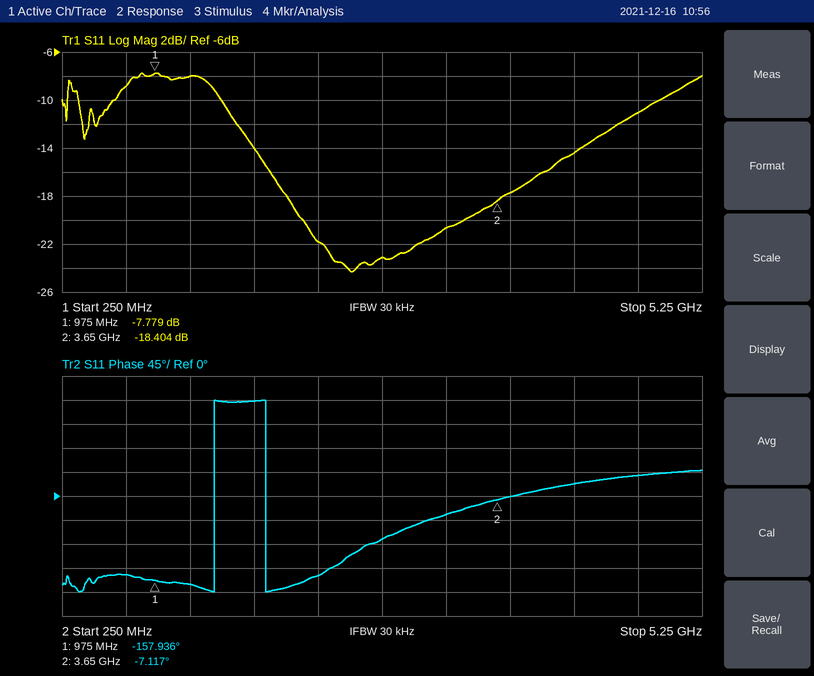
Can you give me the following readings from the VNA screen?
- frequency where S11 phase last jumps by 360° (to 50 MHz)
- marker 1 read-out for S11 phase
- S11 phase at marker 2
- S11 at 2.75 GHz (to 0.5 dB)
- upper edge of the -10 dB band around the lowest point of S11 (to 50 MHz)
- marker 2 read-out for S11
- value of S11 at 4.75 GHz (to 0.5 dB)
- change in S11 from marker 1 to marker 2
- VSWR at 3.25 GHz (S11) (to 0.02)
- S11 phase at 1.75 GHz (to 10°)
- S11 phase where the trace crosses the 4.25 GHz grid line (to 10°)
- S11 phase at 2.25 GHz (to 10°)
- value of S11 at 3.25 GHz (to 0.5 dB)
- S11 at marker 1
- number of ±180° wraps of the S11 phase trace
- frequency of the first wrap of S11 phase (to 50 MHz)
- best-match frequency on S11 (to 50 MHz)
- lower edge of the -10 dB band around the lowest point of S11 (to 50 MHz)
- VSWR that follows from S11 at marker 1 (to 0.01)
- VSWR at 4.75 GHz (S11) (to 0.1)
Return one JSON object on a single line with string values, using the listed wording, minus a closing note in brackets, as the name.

{"frequency where S11 phase last jumps by 360°": "1.85 GHz", "marker 1 read-out for S11 phase": "-157.936°", "S11 phase at marker 2": "-7.117°", "S11 at 2.75 GHz": "-23.0 dB", "upper edge of the -10 dB band around the lowest point of S11": "4.90 GHz", "marker 2 read-out for S11": "-18.404 dB", "value of S11 at 4.75 GHz": "-11.0 dB", "change in S11 from marker 1 to marker 2": "-10.625 dB", "VSWR at 3.25 GHz (S11)": "1.20", "S11 phase at 1.75 GHz": "180°", "S11 phase where the trace crosses the 4.25 GHz grid line": "20°", "S11 phase at 2.25 GHz": "-150°", "value of S11 at 3.25 GHz": "-20.5 dB", "S11 at marker 1": "-7.779 dB", "number of ±180° wraps of the S11 phase trace": "2", "frequency of the first wrap of S11 phase": "1.45 GHz", "best-match frequency on S11": "2.50 GHz", "lower edge of the -10 dB band around the lowest point of S11": "1.50 GHz", "VSWR that follows from S11 at marker 1": "2.38", "VSWR at 4.75 GHz (S11)": "1.8"}
